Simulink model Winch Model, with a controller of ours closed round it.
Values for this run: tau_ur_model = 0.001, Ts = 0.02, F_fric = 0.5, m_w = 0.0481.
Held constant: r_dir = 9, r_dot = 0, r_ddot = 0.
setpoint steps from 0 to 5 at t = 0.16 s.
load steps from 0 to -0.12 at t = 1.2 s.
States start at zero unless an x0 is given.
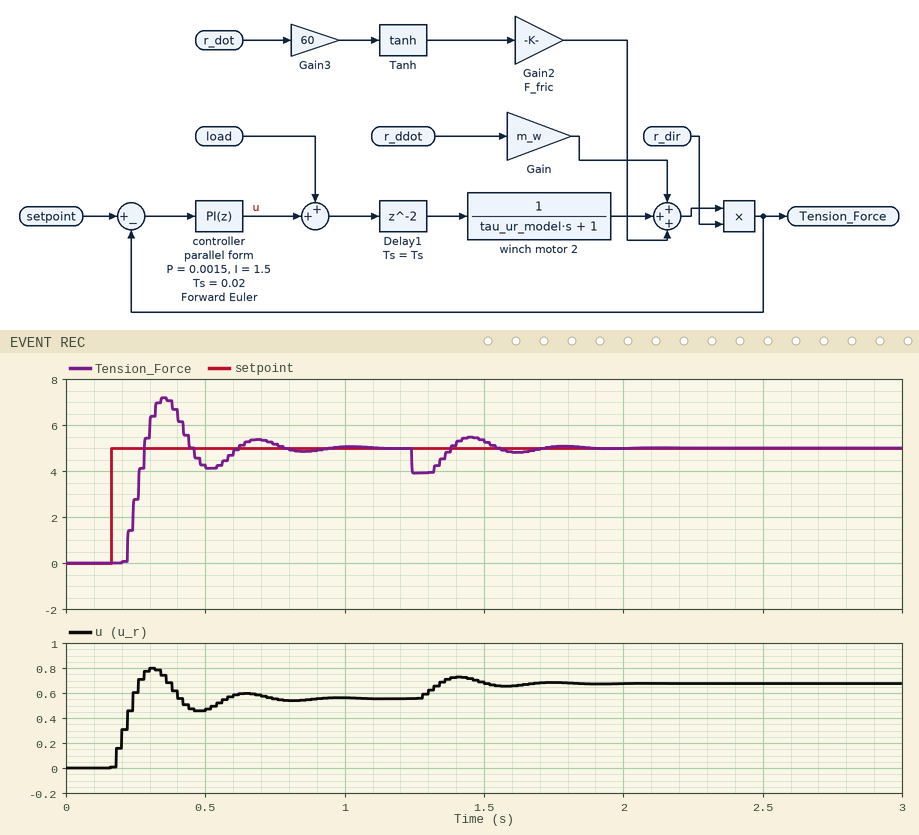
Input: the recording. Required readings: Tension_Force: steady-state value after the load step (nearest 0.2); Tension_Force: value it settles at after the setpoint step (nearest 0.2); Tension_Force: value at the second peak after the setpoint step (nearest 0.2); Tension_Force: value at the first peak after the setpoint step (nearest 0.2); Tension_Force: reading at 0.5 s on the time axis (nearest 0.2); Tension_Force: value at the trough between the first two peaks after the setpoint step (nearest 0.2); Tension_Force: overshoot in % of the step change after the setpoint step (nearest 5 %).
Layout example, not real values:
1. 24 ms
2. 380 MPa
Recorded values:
1. 5.0
2. 5.0
3. 5.4
4. 7.2
5. 4.2
6. 4.2
7. 45 %
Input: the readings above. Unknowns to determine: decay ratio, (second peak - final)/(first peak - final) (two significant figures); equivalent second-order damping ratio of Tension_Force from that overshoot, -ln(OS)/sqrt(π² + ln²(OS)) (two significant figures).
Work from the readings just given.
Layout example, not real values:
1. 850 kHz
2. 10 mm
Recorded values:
1. 0.18
2. 0.25
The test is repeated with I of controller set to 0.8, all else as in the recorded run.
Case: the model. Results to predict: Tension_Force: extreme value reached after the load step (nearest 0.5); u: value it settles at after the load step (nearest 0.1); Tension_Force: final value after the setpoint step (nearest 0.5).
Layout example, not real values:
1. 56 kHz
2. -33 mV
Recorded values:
1. 4.0
2. 0.7
3. 5.0
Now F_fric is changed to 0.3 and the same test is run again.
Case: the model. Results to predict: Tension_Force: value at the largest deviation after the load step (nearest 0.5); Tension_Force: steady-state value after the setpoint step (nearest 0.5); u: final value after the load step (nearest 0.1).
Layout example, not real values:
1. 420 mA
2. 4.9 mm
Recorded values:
1. 4.0
2. 5.0
3. 0.7
